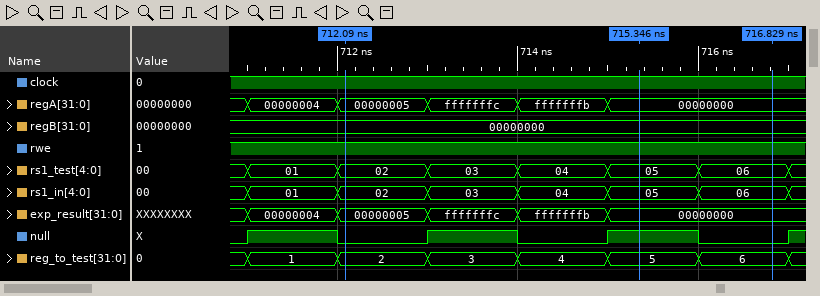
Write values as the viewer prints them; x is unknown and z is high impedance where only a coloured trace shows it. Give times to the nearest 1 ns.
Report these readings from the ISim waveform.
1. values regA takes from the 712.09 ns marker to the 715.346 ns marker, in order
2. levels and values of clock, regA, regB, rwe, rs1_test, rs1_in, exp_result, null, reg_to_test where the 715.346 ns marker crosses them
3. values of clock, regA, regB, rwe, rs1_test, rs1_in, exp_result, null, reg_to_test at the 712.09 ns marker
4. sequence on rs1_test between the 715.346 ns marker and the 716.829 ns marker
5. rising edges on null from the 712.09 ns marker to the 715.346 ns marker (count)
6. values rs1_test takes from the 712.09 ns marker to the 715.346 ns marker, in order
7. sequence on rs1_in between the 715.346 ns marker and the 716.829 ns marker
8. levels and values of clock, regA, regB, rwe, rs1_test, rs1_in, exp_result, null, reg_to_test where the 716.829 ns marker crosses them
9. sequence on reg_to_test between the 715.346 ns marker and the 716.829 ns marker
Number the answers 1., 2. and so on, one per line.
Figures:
1. 00000005, fffffffc, fffffffb, 00000000
2. clock=1, regA=00000000, regB=00000000, rwe=1, rs1_test=05, rs1_in=05, exp_result=00000000, null=1, reg_to_test=5
3. clock=1, regA=00000005, regB=00000000, rwe=1, rs1_test=02, rs1_in=02, exp_result=00000005, null=0, reg_to_test=2
4. 05, 06
5. 2
6. 02, 03, 04, 05
7. 05, 06
8. clock=1, regA=00000000, regB=00000000, rwe=1, rs1_test=06, rs1_in=06, exp_result=00000000, null=0, reg_to_test=6
9. 5, 6
